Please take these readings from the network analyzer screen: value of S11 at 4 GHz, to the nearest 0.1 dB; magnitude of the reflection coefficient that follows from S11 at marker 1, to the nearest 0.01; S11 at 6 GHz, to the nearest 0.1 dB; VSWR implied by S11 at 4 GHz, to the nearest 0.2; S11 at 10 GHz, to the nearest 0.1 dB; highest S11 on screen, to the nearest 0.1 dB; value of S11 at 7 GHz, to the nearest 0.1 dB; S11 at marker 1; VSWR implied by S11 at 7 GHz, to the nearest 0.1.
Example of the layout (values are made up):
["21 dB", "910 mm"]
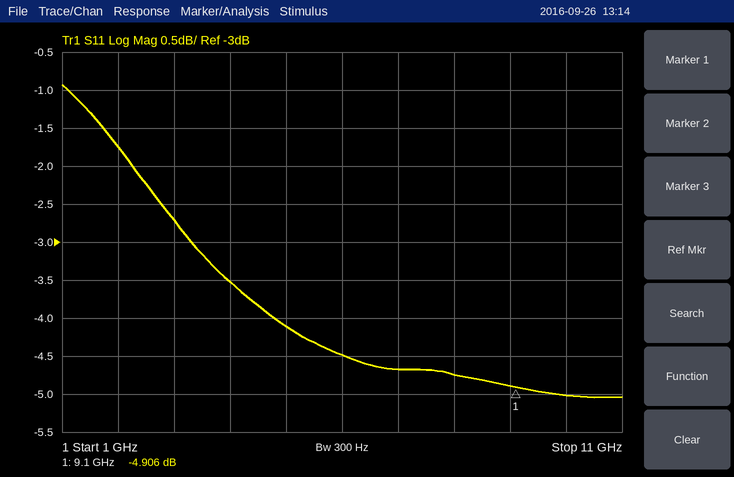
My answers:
["-3.5 dB", "0.57", "-4.5 dB", "5.0", "-5.0 dB", "-0.9 dB", "-4.7 dB", "-4.906 dB", "3.8"]
